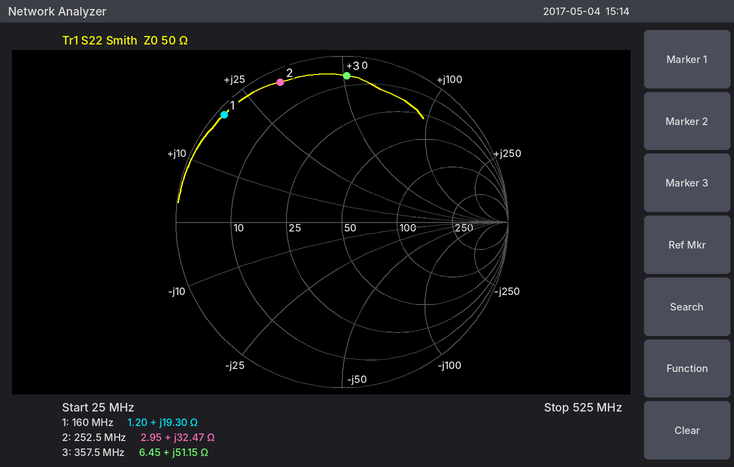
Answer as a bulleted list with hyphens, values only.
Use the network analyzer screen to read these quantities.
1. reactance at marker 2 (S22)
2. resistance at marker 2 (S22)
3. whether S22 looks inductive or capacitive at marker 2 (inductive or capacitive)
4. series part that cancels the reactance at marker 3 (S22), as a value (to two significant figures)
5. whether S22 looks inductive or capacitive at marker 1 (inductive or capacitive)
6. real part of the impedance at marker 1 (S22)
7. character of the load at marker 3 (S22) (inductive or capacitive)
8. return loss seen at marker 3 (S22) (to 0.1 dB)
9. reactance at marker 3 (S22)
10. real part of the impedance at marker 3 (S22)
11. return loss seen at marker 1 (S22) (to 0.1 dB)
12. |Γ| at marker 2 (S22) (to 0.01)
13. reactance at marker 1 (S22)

- +32.47 Ω
- 2.95 Ω
- inductive
- 8.7 pF
- inductive
- 1.20 Ω
- inductive
- 1.1 dB
- +51.15 Ω
- 6.45 Ω
- 0.4 dB
- 0.92
- +19.30 Ω
